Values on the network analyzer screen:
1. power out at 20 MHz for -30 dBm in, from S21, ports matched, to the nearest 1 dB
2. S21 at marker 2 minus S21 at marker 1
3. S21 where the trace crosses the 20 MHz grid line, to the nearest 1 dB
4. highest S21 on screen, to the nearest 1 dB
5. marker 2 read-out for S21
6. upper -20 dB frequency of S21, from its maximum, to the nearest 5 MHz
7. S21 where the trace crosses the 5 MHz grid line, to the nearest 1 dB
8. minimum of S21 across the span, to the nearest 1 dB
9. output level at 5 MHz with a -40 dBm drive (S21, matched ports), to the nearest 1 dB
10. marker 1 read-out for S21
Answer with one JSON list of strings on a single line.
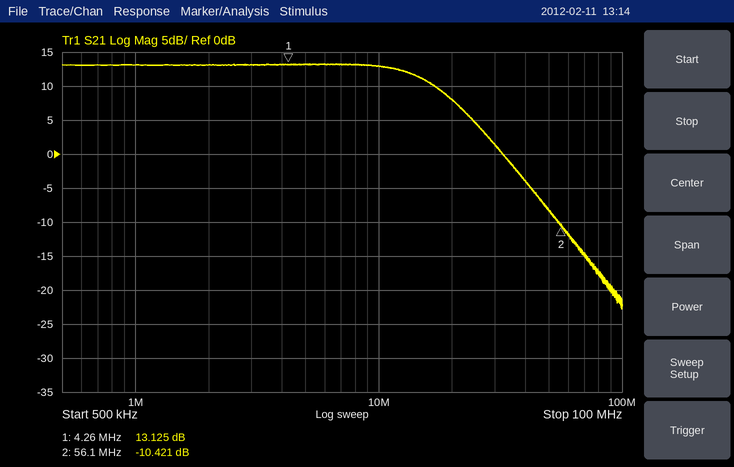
["-22 dBm", "-23.546 dB", "8 dB", "13 dB", "-10.421 dB", "45 MHz", "13 dB", "-23 dB", "-27 dBm", "13.125 dB"]
